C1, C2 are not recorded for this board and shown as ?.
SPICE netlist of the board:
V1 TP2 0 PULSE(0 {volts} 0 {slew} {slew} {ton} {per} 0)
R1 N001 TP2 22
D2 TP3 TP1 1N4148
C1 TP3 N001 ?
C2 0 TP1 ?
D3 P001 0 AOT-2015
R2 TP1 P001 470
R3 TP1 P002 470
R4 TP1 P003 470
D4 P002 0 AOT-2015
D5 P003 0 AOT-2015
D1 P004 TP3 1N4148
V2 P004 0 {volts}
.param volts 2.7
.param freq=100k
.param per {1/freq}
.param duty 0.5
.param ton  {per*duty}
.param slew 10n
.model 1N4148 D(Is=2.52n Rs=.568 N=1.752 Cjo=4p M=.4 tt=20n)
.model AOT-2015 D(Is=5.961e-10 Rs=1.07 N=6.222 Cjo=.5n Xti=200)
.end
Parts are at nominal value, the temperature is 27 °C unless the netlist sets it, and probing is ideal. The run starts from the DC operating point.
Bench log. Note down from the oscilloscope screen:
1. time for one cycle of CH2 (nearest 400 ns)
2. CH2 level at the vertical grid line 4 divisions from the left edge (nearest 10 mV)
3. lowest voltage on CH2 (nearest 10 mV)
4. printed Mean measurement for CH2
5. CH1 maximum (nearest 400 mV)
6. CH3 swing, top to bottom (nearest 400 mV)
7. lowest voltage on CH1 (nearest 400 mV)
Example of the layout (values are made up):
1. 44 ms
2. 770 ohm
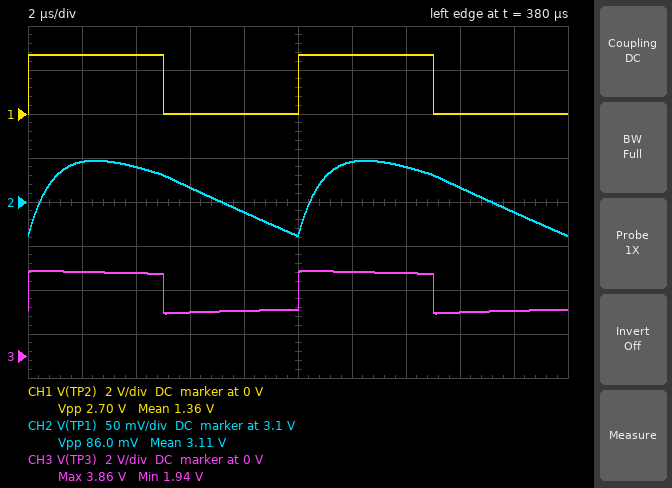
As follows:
1. 10.0 µs
2. 3.09 V
3. 3.06 V
4. 3.11 V
5. 2.8 V
6. 2.0 V
7. 0 V
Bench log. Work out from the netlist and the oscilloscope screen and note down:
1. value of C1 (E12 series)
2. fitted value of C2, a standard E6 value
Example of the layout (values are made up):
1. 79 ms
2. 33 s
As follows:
1. 47 nF
2. 330 nF
